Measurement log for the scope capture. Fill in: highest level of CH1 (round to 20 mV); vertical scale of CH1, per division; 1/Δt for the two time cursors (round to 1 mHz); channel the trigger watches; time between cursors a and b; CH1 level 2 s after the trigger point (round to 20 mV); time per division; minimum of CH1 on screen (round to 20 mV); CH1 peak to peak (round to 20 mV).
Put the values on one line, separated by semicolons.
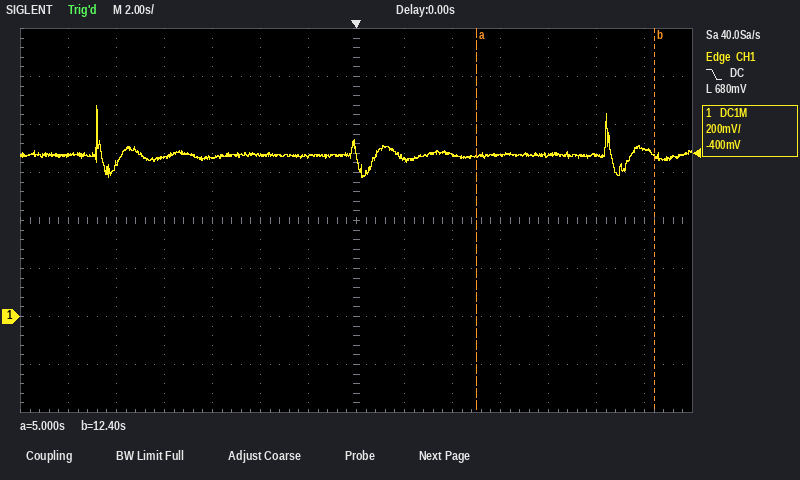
880 mV; 200 mV; 135 mHz; CH1; 7.4 s; 660 mV; 2 s; 580 mV; 300 mV
